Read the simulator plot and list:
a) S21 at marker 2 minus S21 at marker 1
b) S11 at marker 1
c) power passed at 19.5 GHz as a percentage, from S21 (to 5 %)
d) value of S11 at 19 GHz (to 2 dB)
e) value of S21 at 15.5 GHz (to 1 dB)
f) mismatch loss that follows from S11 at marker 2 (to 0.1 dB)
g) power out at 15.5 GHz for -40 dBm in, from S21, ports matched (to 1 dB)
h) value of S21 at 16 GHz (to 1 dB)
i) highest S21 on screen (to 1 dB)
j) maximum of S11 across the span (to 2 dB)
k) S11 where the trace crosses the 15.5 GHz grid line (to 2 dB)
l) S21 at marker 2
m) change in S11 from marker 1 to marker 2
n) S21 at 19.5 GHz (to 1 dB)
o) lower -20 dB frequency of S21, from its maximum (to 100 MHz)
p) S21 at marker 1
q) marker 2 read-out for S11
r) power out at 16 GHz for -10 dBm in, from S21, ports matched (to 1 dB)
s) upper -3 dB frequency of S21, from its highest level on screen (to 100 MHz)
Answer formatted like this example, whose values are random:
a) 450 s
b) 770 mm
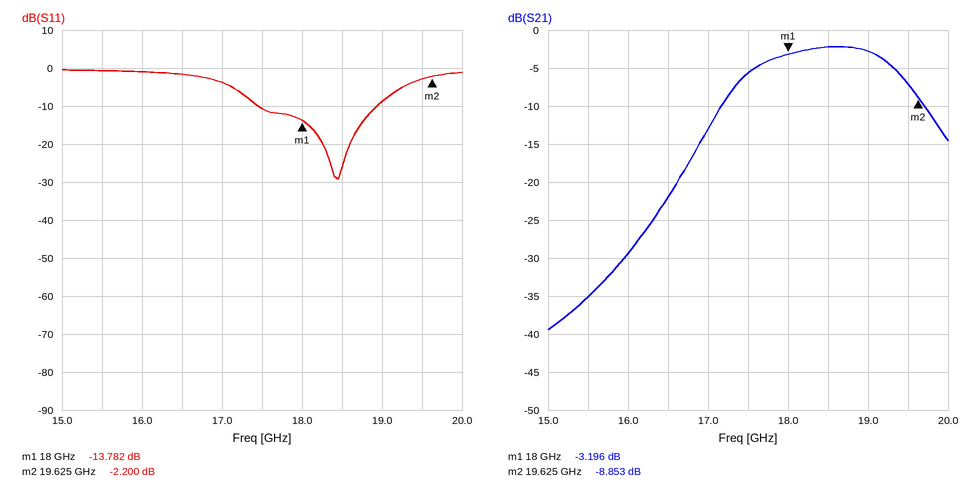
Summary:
a) -5.657 dB
b) -13.782 dB
c) 20 %
d) -8 dB
e) -35 dB
f) 4.0 dB
g) -75 dBm
h) -29 dB
i) -2 dB
j) 0 dB
k) 0 dB
l) -8.853 dB
m) 11.582 dB
n) -7 dB
o) 16.5 GHz
p) -3.196 dB
q) -2.200 dB
r) -39 dBm
s) 19.3 GHz
